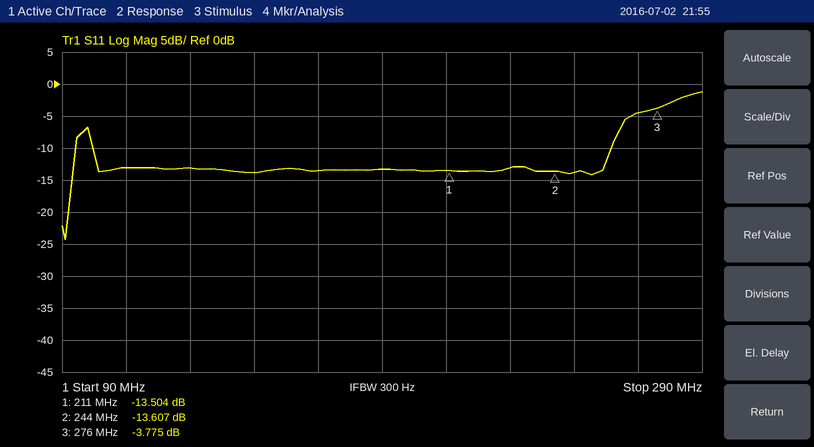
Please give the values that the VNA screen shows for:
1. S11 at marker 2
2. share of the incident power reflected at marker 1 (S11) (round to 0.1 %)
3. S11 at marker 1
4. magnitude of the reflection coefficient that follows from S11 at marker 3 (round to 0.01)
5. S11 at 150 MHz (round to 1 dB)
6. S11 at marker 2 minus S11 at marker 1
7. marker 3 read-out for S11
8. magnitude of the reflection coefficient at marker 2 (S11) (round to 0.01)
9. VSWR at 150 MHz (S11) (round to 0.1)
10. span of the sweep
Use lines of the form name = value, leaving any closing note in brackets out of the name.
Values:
S11 at marker 2 = -13.607 dB
share of the incident power reflected at marker 1 (S11) = 4.5 %
S11 at marker 1 = -13.504 dB
magnitude of the reflection coefficient that follows from S11 at marker 3 = 0.65
S11 at 150 MHz = -14 dB
S11 at marker 2 minus S11 at marker 1 = -0.103 dB
marker 3 read-out for S11 = -3.775 dB
magnitude of the reflection coefficient at marker 2 (S11) = 0.21
VSWR at 150 MHz (S11) = 1.5
span of the sweep = 200 MHz
